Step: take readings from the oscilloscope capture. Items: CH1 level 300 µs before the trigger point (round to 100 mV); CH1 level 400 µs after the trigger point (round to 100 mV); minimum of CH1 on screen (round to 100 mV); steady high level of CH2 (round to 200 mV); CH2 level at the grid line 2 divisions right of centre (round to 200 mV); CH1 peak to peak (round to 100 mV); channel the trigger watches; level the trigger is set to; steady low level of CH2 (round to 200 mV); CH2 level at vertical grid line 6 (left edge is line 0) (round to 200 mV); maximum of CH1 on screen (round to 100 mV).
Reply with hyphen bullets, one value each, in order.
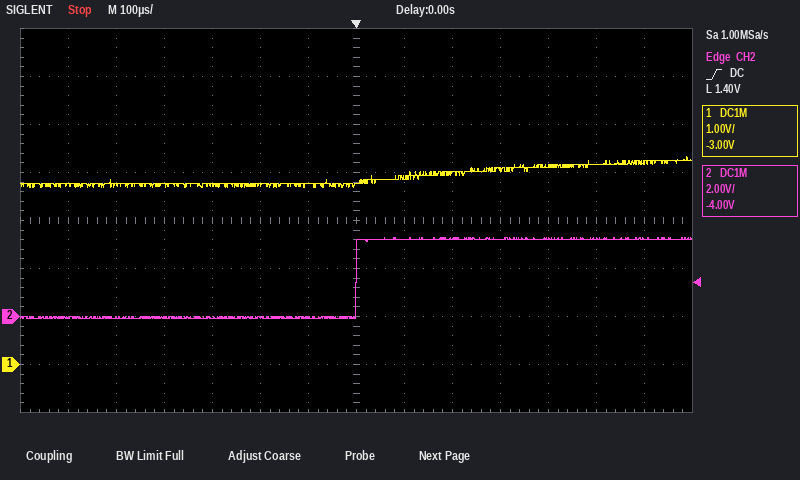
- 3.7 V
- 4.1 V
- 3.7 V
- 3.2 V
- 3.2 V
- 600 mV
- CH2
- 1.40 V
- 0.0 V
- 0.0 V
- 4.3 V
